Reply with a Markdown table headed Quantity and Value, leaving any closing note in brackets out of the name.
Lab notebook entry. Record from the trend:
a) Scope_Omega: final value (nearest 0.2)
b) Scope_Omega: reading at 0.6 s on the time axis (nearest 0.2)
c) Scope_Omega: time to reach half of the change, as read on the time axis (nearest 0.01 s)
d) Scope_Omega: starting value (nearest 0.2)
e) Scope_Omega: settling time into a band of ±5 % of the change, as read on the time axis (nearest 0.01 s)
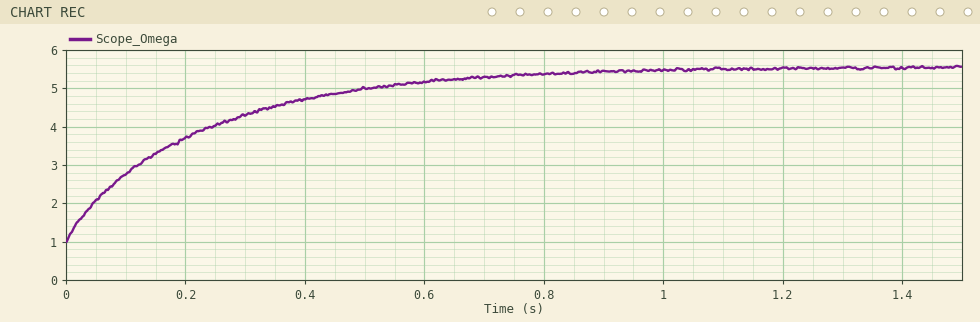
| Quantity | Value |
|---|---|
| Scope_Omega: final value | 5.6 |
| Scope_Omega: reading at 0.6 s on the time axis | 5.2 |
| Scope_Omega: time to reach half of the change, as read on the time axis | 0.15 s |
| Scope_Omega: starting value | 1.0 |
| Scope_Omega: settling time into a band of ±5 % of the change, as read on the time axis | 0.74 s |
